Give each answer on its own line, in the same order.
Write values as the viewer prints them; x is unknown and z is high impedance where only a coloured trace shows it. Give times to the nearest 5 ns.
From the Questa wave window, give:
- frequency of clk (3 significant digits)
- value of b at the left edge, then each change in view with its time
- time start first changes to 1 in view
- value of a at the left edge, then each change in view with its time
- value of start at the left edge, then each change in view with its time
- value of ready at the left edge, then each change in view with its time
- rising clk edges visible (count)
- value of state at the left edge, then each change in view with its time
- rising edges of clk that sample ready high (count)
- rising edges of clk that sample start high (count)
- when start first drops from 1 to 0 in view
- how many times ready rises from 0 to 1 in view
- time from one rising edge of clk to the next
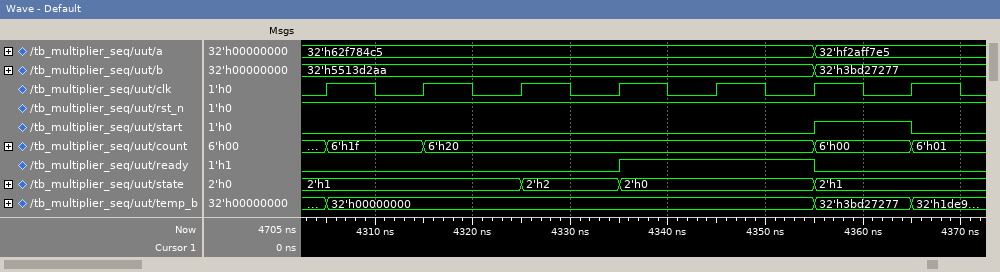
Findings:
100 MHz
32'h5513d2aa, 32'h3bd27277 at 4355 ns
4355 ns
32'h62f784c5, 32'hf2aff7e5 at 4355 ns
0, 1 at 4355 ns, 0 at 4365 ns
0, 1 at 4335 ns, 0 at 4355 ns
7
2'h1, 2'h2 at 4325 ns, 2'h0 at 4335 ns, 2'h1 at 4355 ns
2
1
4365 ns
1
10 ns
